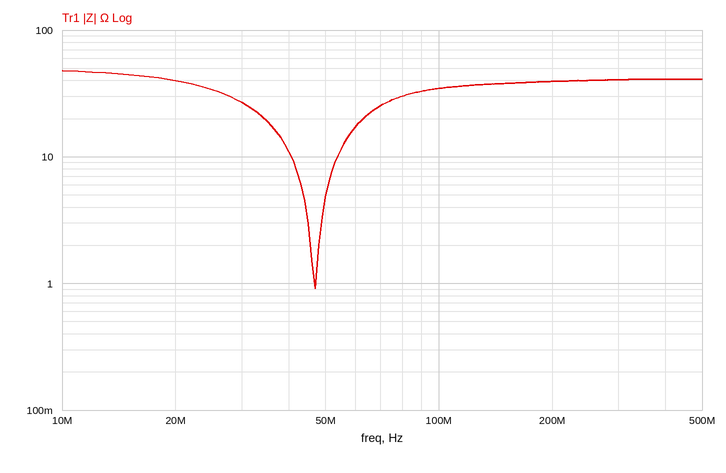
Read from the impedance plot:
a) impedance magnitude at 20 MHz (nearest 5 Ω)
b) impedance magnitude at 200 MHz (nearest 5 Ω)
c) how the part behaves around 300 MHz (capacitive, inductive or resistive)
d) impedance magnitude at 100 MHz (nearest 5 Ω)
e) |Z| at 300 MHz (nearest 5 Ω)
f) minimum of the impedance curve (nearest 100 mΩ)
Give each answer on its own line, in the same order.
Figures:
40 Ω
40 Ω
resistive
35 Ω
40 Ω
900 mΩ
